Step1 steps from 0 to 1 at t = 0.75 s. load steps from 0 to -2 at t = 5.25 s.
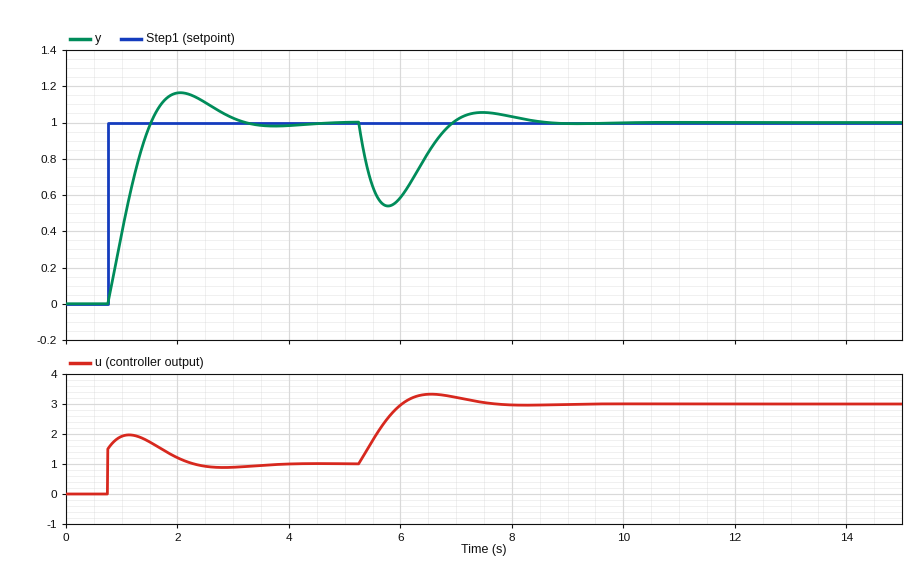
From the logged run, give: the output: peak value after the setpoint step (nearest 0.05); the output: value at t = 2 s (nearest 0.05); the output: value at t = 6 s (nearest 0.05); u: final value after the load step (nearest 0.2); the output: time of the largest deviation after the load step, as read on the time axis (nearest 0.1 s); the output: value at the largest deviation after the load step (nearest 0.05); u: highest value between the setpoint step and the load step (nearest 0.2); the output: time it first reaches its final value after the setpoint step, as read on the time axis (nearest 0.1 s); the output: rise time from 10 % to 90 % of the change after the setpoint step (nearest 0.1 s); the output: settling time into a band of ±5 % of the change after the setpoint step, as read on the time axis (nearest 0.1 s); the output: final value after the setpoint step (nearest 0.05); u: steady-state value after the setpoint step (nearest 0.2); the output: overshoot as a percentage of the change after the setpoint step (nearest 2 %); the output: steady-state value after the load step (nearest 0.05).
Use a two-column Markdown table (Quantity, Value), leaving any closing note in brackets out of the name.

| Quantity | Value |
|---|---|
| the output: peak value after the setpoint step | 1.15 |
| the output: value at t = 2 s | 1.15 |
| the output: value at t = 6 s | 0.60 |
| u: final value after the load step | 3.0 |
| the output: time of the largest deviation after the load step, as read on the time axis | 5.8 s |
| the output: value at the largest deviation after the load step | 0.55 |
| u: highest value between the setpoint step and the load step | 2.0 |
| the output: time it first reaches its final value after the setpoint step, as read on the time axis | 1.5 s |
| the output: rise time from 10 % to 90 % of the change after the setpoint step | 0.6 s |
| the output: settling time into a band of ±5 % of the change after the setpoint step, as read on the time axis | 2.8 s |
| the output: final value after the setpoint step | 1.00 |
| u: steady-state value after the setpoint step | 1.0 |
| the output: overshoot as a percentage of the change after the setpoint step | 16 % |
| the output: steady-state value after the load step | 1.00 |
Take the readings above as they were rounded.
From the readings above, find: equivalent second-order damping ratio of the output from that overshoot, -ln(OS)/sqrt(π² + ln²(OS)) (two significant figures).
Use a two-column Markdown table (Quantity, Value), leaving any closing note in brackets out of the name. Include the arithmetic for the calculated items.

| Quantity | Value |
|---|---|
| equivalent second-order damping ratio of the output from that overshoot, -ln(OS)/sqrt(π² + ln²(OS)) | ln(0.16) = -1.833; 1.833 / sqrt(9.870 + 3.358) = 0.50 |
